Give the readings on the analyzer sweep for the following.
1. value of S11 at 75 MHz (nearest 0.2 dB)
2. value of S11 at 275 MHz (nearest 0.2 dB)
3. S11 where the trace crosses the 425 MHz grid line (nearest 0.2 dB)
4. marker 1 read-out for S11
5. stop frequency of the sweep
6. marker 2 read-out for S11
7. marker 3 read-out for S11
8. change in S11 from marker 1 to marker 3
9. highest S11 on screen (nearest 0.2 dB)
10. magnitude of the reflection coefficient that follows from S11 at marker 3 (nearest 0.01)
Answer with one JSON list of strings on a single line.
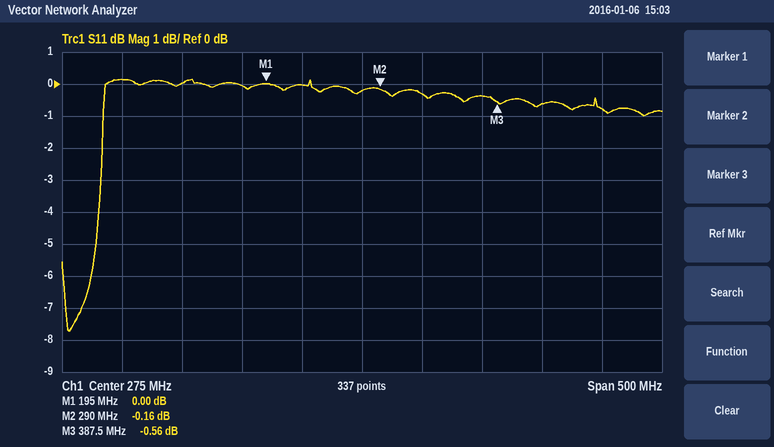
["0.2 dB", "-0.2 dB", "-0.6 dB", "0.00 dB", "525 MHz", "-0.16 dB", "-0.56 dB", "-0.56 dB", "0.2 dB", "0.94"]
